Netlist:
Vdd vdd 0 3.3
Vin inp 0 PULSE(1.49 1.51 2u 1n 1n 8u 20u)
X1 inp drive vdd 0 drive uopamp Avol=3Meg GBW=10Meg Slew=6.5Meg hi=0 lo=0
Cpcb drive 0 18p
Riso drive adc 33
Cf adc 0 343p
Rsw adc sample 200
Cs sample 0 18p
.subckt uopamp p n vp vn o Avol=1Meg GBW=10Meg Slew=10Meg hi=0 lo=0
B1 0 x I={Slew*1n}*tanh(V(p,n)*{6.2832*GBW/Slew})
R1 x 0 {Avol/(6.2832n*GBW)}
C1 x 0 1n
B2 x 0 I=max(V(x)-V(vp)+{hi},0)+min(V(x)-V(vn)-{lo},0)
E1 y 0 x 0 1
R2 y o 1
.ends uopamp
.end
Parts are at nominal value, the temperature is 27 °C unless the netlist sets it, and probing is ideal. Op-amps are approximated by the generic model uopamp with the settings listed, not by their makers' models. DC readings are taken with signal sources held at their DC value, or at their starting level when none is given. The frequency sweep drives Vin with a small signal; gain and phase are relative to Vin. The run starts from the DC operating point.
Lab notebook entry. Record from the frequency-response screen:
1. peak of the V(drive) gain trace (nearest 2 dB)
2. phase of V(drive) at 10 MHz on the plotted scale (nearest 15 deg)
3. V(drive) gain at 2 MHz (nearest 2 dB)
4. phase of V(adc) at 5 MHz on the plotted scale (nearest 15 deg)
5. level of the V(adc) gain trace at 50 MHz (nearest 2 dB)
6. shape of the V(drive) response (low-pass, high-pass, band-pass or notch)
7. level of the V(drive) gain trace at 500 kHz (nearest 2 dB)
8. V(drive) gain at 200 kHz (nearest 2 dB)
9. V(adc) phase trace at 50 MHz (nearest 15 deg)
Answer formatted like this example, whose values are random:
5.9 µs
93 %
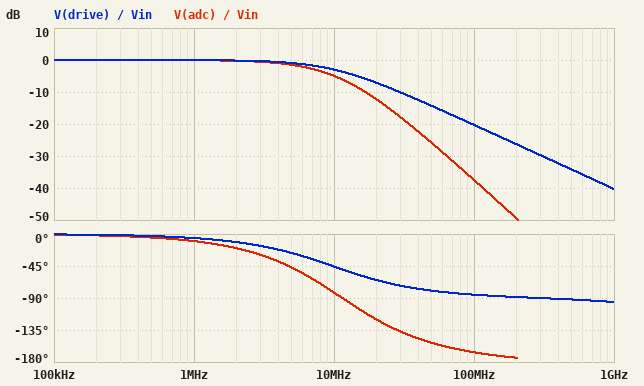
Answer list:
0 dB
-45 deg
0 dB
-45 deg
-26 dB
low-pass
0 dB
0 dB
-150 deg
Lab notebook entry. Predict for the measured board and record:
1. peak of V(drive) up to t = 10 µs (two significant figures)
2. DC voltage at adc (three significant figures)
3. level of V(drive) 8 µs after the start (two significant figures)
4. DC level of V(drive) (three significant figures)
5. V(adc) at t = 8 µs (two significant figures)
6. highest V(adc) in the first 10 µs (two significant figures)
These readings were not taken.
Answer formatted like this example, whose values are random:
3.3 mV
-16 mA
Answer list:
1.5 V
1.49 V
1.5 V
1.49 V
1.5 V
1.5 V
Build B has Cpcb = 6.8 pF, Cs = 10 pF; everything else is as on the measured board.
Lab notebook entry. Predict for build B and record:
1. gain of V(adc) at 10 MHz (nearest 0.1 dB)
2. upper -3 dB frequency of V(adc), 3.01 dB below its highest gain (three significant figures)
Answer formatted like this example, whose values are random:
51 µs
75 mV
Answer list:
-4.9 dB
7.43 MHz
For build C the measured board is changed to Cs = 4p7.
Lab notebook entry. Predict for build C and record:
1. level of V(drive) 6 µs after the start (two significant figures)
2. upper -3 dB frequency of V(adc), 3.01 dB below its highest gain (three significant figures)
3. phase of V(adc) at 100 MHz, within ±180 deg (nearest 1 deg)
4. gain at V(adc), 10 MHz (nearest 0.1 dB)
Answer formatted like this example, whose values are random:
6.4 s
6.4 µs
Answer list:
1.5 V
7.49 MHz
-167 deg
-4.8 dB
